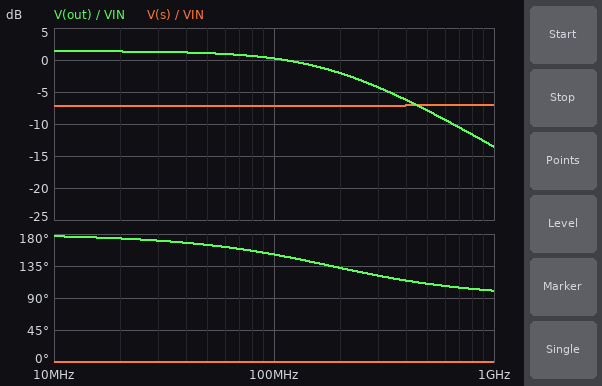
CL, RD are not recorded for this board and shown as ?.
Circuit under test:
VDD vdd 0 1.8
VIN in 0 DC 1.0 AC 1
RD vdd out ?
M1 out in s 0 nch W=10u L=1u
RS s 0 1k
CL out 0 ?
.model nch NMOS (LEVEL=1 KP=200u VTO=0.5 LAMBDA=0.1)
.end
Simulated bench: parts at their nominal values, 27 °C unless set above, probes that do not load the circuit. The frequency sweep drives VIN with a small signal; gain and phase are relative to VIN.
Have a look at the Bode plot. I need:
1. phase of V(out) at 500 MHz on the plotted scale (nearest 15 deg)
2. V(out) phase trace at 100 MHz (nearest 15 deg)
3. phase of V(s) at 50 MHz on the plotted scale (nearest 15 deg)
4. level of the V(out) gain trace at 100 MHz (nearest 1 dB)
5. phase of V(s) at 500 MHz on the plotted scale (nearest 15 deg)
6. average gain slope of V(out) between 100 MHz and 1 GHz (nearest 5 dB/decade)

105 deg
150 deg
0 deg
0 dB
0 deg
-15 dB/decade
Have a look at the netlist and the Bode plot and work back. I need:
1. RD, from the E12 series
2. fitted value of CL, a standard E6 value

2.7 kΩ
330 fF
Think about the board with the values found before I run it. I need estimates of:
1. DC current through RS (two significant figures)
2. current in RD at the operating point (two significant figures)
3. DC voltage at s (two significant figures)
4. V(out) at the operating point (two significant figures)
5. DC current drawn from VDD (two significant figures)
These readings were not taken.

140 µA
140 µA
140 mV
1.4 V
140 µA
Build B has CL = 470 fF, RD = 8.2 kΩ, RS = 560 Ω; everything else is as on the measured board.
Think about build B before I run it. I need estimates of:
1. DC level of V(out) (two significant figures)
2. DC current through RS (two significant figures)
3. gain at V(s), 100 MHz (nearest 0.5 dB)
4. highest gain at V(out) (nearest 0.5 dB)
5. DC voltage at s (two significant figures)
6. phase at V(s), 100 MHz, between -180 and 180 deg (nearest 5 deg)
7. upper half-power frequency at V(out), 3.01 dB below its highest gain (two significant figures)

430 mV
170 µA
-13.0 dB
6.5 dB
93 mV
15 deg
76 MHz
